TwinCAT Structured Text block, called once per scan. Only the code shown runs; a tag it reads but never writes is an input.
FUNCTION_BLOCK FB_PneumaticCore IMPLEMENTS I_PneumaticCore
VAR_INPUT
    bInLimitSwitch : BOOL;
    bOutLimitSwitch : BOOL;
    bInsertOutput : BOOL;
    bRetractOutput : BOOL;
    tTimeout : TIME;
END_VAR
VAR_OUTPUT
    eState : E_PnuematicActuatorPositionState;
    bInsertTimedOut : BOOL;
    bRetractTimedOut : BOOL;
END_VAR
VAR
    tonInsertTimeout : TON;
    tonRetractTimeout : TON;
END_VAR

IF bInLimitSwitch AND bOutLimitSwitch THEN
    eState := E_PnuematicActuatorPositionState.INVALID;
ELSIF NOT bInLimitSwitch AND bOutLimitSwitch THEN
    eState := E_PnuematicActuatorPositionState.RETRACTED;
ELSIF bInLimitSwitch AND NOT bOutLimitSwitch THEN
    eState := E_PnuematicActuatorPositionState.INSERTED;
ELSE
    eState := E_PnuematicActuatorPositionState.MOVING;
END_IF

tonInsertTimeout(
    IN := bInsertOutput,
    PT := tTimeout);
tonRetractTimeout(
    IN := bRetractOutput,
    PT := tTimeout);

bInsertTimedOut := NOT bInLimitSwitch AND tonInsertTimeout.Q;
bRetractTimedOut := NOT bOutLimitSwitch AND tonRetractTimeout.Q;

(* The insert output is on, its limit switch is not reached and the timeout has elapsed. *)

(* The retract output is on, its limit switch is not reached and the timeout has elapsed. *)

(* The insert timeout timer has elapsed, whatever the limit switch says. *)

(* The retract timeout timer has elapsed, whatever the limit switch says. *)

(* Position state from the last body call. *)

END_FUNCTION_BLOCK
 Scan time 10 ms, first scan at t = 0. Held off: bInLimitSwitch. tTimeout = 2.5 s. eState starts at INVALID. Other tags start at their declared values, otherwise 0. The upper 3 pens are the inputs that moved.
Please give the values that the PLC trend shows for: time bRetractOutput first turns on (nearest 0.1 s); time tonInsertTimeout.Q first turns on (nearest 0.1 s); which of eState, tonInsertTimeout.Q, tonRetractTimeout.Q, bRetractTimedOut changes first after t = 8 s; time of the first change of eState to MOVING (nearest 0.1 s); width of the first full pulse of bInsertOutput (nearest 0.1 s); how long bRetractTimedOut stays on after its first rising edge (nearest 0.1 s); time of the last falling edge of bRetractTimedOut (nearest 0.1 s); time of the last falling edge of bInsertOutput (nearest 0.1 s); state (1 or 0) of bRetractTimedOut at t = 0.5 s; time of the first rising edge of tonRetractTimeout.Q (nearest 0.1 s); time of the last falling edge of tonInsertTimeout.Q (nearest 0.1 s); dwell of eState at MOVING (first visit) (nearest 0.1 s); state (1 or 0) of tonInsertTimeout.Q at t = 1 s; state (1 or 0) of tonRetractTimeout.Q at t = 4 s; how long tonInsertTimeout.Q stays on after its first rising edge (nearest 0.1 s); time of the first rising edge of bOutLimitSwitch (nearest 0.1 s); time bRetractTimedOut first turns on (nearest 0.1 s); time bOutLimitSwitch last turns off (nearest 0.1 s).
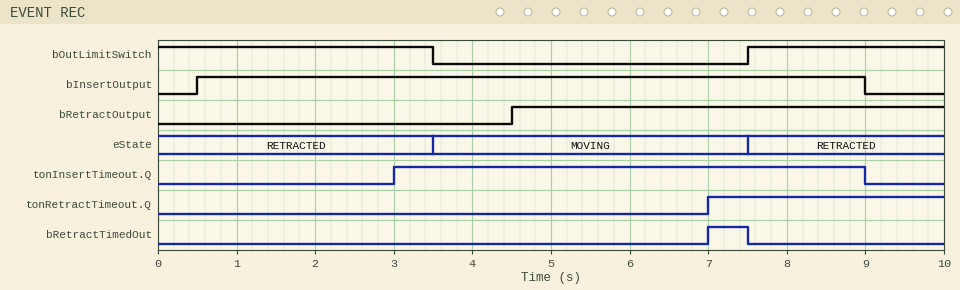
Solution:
4.5 s
3.0 s
tonInsertTimeout.Q
3.5 s
8.5 s
0.5 s
7.5 s
9.0 s
0
7.0 s
9.0 s
4.0 s
0
0
6.0 s
7.5 s
7.0 s
3.5 s
